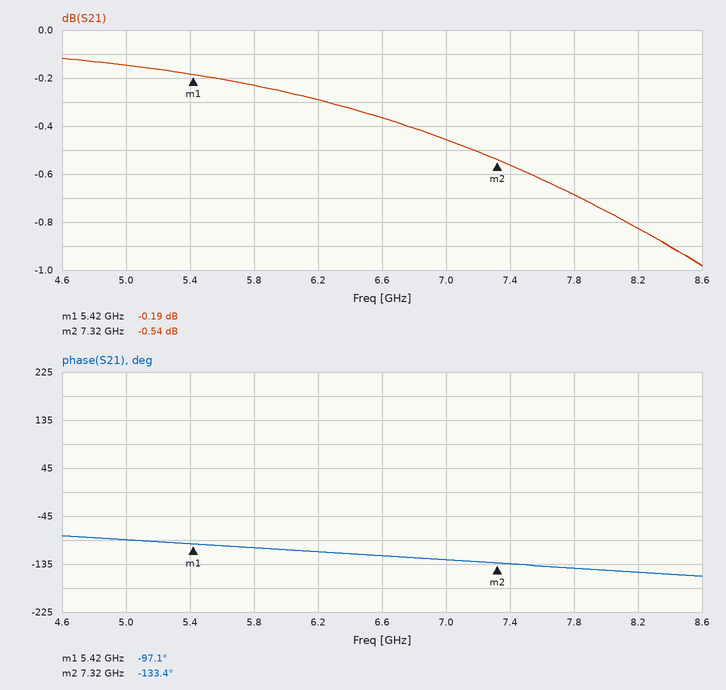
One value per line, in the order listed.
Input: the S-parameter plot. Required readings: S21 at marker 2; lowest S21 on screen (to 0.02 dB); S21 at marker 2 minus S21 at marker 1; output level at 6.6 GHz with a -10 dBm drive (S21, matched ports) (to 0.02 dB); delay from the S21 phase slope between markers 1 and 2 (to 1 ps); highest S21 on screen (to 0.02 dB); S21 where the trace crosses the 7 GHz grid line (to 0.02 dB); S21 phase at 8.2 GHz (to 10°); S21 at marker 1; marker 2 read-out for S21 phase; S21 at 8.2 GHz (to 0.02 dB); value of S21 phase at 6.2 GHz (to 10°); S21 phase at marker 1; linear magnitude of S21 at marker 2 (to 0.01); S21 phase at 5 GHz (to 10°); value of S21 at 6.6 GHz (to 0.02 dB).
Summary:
-0.54 dB
-0.98 dB
-0.35 dB
-10.36 dBm
53 ps
-0.12 dB
-0.46 dB
-150°
-0.19 dB
-133.4°
-0.82 dB
-110°
-97.1°
0.94
-90°
-0.36 dB
